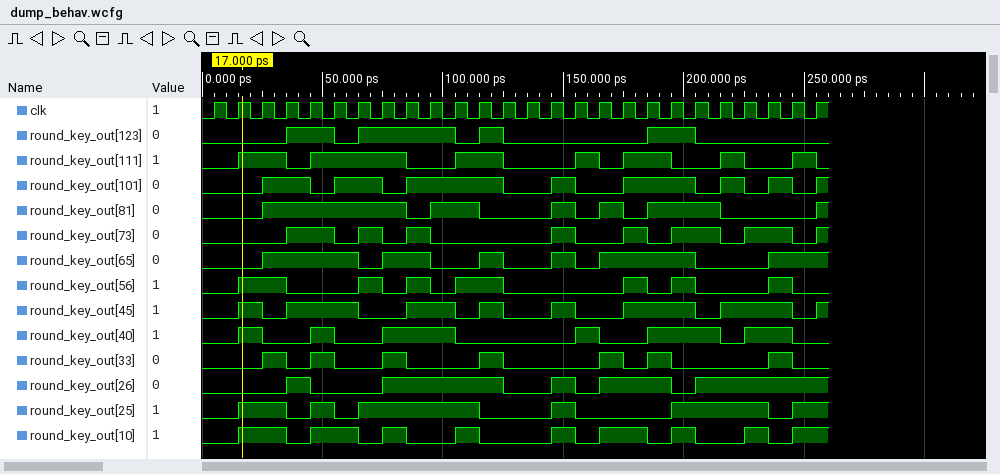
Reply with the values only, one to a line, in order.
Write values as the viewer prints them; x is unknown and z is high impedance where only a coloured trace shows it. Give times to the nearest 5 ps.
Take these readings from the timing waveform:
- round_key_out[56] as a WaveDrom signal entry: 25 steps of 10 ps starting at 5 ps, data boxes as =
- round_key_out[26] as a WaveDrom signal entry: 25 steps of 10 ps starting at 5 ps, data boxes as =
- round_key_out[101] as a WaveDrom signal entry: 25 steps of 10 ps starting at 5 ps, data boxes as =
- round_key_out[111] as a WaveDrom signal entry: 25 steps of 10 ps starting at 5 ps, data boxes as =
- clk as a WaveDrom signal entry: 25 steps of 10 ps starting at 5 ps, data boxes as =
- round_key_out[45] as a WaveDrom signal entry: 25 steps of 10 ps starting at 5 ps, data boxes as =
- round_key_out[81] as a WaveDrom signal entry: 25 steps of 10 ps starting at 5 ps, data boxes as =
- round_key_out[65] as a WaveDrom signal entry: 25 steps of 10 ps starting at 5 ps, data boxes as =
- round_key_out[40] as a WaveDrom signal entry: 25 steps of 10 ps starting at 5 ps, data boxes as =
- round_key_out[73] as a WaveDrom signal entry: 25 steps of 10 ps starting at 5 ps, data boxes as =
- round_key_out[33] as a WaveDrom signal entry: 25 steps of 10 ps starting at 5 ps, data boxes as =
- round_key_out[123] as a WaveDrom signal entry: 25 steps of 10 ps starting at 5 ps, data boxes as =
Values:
{name: 'round_key_out[56]', wave: '01.0..10101.0....1010..10'}
{name: 'round_key_out[26]', wave: '0..10..1....0.101..01....'}
{name: 'round_key_out[101]', wave: '0.1.01.01...0.10.1..01010'}
{name: 'round_key_out[111]', wave: '01.01...0.1.0..101.0.10.1'}
{name: 'clk', wave: 'p........................'}
{name: 'round_key_out[45]', wave: '0101..0.1.010.10.1..01..0'}
{name: 'round_key_out[81]', wave: '0.1.....01.0..10101..0...'}
{name: 'round_key_out[65]', wave: '0.1...01.0.10.101...0..1.'}
{name: 'round_key_out[40]', wave: '010.10.1..0....10.1..01.0'}
{name: 'round_key_out[73]', wave: '0..1.01010....10.101.01.0'}
{name: 'round_key_out[33]', wave: '0.1010.10..10...1010...10'}
{name: 'round_key_out[123]', wave: '0..1.01...010.....1.0....'}
